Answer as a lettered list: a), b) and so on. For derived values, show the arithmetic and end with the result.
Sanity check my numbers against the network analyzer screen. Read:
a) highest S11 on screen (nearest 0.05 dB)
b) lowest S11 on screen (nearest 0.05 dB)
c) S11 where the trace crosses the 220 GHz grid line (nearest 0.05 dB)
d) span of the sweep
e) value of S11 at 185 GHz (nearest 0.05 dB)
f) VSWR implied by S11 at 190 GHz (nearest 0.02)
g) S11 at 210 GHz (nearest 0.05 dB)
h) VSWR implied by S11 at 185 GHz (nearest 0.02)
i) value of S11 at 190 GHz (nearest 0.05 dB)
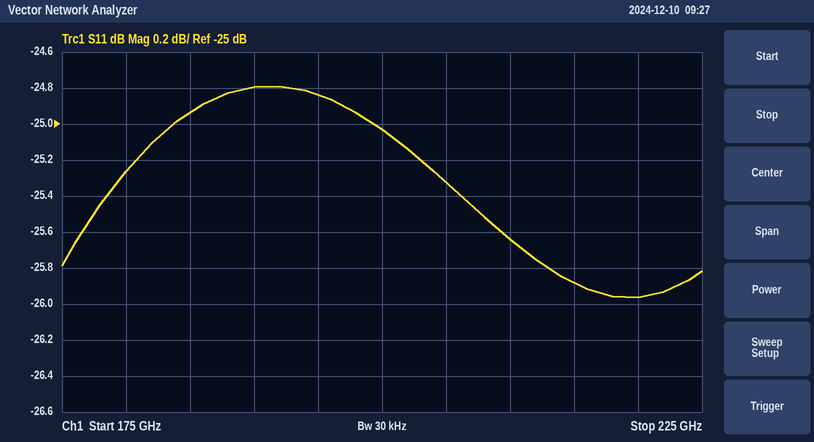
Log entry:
a) -24.80 dB
b) -25.95 dB
c) -25.95 dB
d) 50 GHz
e) -24.95 dB
f) |Γ| = 10^(-24.8/20) = 0.0575; VSWR = (1 + 0.0575)/(1 − 0.0575) ≈ 1.12
g) -25.65 dB
h) |Γ| = 10^(-24.95/20) = 0.0566; VSWR = (1 + 0.0566)/(1 − 0.0566) ≈ 1.12
i) -24.80 dB
